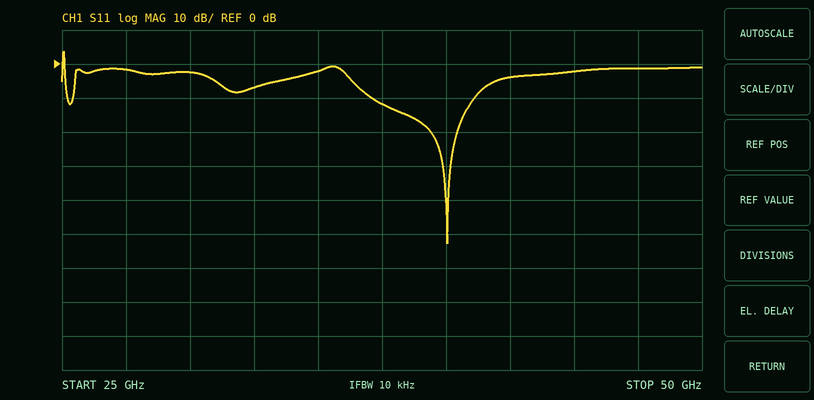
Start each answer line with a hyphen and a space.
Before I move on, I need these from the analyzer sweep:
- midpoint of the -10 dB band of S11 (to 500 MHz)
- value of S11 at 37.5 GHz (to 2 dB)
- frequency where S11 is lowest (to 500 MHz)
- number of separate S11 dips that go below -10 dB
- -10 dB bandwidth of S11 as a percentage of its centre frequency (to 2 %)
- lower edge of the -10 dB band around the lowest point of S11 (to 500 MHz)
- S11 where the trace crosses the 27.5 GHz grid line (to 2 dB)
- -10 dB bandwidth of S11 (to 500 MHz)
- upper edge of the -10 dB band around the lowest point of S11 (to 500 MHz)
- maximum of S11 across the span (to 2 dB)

- 39.0 GHz
- -12 dB
- 40.0 GHz
- 2
- 10 %
- 37.0 GHz
- -2 dB
- 4.0 GHz
- 41.0 GHz
- 4 dB
